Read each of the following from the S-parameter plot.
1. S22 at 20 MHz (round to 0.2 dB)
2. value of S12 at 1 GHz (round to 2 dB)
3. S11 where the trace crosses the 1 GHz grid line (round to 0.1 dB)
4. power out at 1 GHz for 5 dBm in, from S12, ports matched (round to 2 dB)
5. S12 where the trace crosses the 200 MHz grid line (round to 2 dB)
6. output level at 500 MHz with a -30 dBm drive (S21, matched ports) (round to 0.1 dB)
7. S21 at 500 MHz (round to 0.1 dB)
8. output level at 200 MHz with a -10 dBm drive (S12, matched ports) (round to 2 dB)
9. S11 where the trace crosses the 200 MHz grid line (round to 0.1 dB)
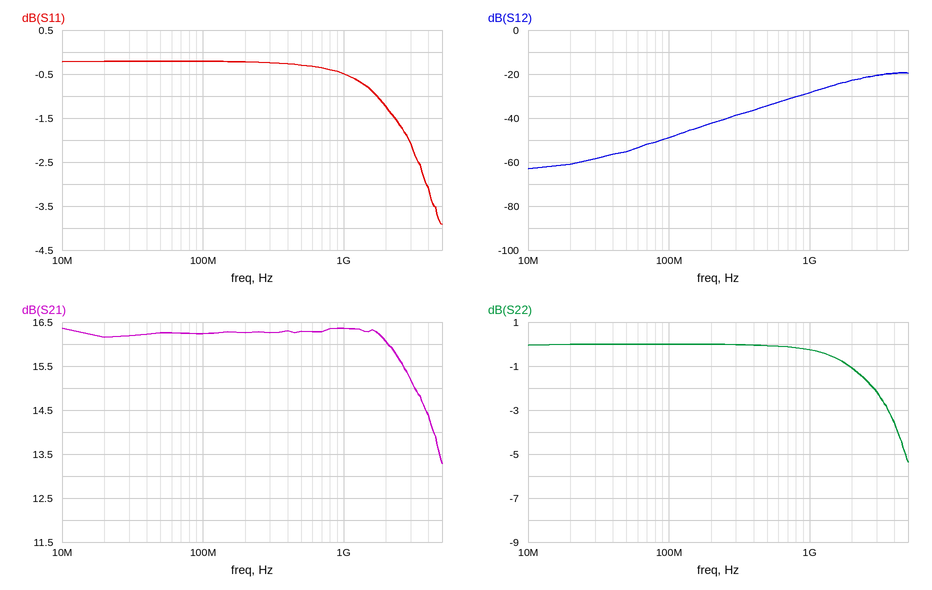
0.0 dB
-28 dB
-0.5 dB
-24 dBm
-42 dB
-13.7 dBm
16.3 dB
-52 dBm
-0.2 dB
